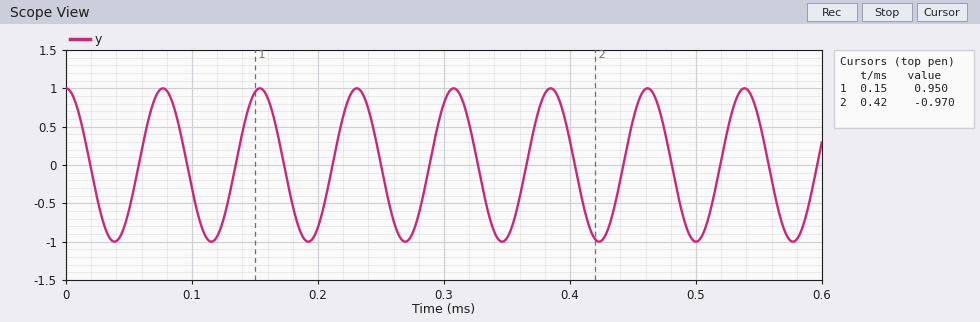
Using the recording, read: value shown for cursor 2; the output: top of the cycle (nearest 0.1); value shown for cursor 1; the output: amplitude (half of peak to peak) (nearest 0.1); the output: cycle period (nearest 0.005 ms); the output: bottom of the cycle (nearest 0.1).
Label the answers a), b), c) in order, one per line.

a) -0.970
b) 1.0
c) 0.950
d) 1.0
e) 0.075 ms
f) -1.0
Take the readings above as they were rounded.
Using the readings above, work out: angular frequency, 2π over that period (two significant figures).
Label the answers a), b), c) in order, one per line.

a) 84 rad/ms
